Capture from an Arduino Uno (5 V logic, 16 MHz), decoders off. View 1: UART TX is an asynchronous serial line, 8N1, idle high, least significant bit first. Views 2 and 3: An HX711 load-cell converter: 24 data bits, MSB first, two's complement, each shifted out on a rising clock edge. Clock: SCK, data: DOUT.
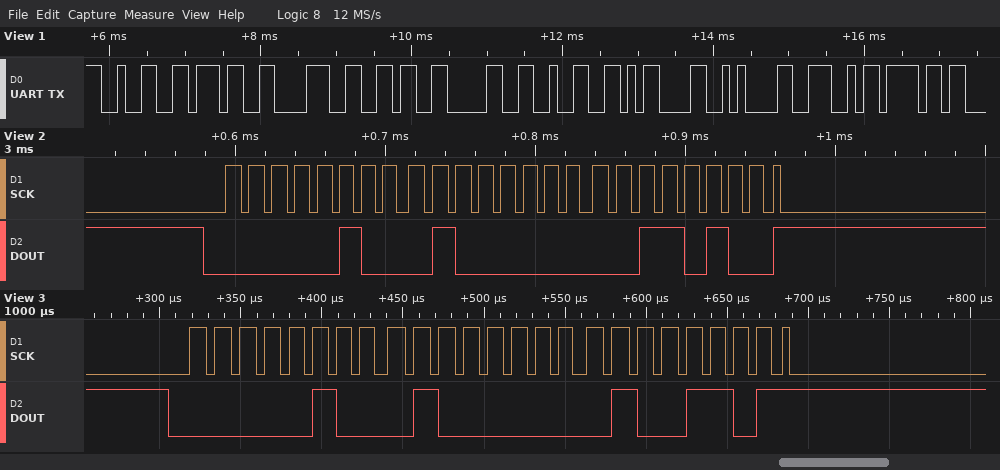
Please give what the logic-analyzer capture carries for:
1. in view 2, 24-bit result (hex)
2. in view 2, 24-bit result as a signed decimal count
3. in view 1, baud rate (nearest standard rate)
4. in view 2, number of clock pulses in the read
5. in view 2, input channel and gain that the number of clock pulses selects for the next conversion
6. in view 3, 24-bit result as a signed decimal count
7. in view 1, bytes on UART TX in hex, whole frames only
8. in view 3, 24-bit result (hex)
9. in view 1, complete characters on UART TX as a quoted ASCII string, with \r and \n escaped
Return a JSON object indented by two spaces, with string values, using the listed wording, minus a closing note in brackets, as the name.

{
  "in view 2, 24-bit result": "0x044034",
  "in view 2, 24-bit result as a signed decimal count": "278580",
  "in view 1, baud rate": "9600 baud",
  "in view 2, number of clock pulses in the read": "25",
  "in view 2, input channel and gain that the number of clock pulses selects for the next conversion": "channel A, gain 128",
  "in view 3, 24-bit result as a signed decimal count": "278605",
  "in view 1, bytes on UART TX in hex, whole frames only": "32 37 38 36 30 32 0D 0A 4E 6F",
  "in view 3, 24-bit result": "0x04404D",
  "in view 1, complete characters on UART TX as a quoted ASCII string, with \\r and \\n escaped": "\"278602\\r\\nNo\""
}
